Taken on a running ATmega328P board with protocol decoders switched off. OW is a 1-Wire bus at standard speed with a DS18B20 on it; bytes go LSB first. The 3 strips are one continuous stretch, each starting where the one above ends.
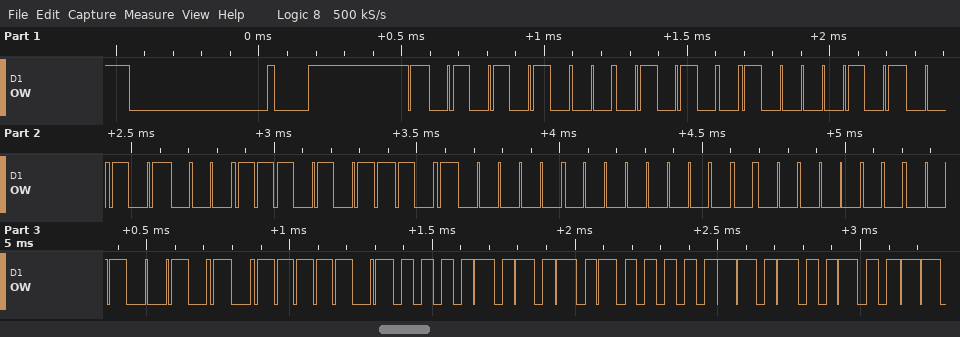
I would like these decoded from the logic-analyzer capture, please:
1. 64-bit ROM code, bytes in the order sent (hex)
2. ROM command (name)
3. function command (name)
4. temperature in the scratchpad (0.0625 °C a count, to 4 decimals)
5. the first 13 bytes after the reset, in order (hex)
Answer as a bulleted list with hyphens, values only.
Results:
- 28 A1 14 D7 05 00 00 A4
- Match ROM
- Read Scratchpad
- 85.0000 °C
- 55 28 A1 14 D7 05 00 00 A4 BE 50 05 4B
